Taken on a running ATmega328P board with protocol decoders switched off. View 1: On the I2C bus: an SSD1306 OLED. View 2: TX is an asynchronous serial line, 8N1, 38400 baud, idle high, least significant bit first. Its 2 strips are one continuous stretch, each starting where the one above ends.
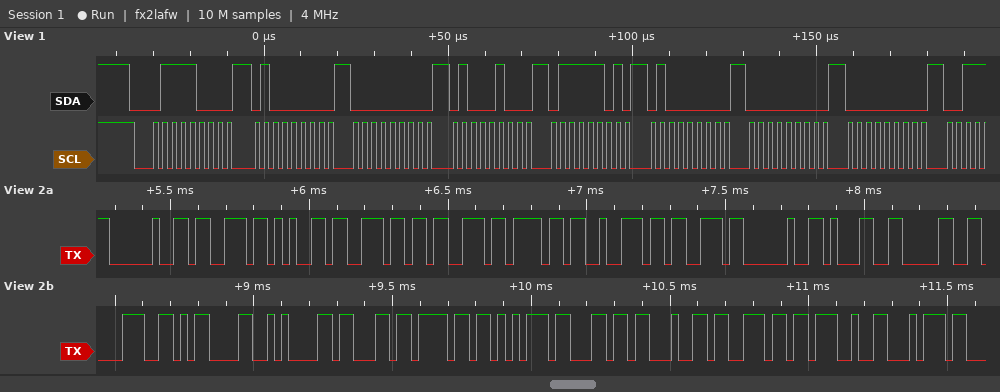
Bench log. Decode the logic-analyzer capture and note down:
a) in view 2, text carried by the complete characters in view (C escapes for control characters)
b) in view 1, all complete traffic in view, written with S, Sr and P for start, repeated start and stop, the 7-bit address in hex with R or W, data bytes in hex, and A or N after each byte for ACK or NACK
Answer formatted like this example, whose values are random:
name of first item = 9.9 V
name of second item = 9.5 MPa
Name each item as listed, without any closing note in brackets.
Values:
in view 2, text carried by the complete characters in view = " sensors 108\r\ncouldn't"
in view 1, all complete traffic in view, written with S, Sr and P for start, repeated start and stop, the 7-bit address in hex with R or W, data bytes in hex, and A or N after each byte for ACK or NACK = S 3CW A 40 A 00 A 44 A 7D A 40 A 00 A 00 A
